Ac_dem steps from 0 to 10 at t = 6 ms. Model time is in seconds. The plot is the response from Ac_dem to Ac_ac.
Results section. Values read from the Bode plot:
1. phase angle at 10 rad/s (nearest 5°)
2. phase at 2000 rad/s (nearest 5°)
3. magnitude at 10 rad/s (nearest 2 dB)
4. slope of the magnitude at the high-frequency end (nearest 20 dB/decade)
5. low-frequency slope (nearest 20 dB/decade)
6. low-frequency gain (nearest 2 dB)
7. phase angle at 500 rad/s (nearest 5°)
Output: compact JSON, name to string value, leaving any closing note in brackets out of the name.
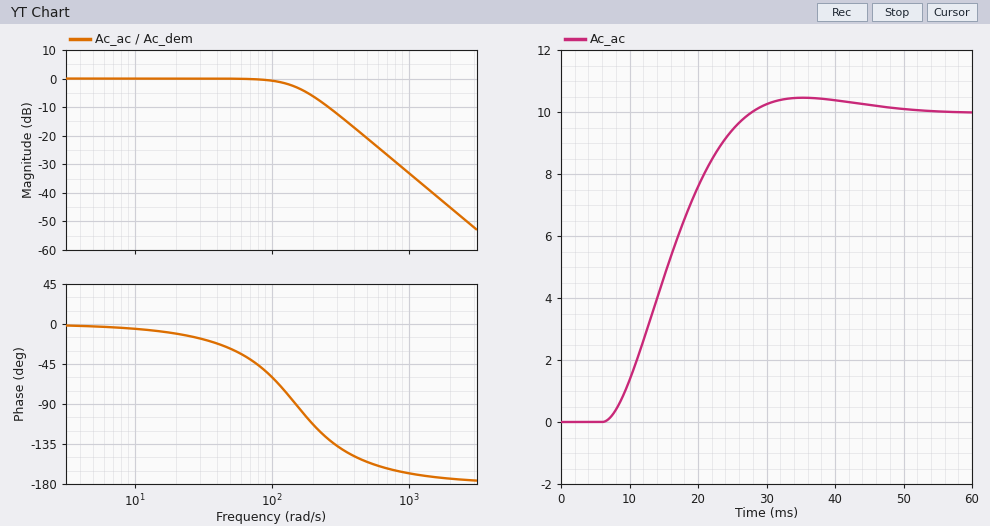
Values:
{"phase angle at 10 rad/s": "-5°", "phase at 2000 rad/s": "-175°", "magnitude at 10 rad/s": "0 dB", "slope of the magnitude at the high-frequency end": "-40 dB/decade", "low-frequency slope": "0 dB/decade", "low-frequency gain": "0 dB", "phase angle at 500 rad/s": "-155°"}
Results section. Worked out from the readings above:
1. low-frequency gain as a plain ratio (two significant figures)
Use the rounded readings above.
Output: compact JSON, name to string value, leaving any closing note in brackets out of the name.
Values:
{"low-frequency gain as a plain ratio": "1.0"}
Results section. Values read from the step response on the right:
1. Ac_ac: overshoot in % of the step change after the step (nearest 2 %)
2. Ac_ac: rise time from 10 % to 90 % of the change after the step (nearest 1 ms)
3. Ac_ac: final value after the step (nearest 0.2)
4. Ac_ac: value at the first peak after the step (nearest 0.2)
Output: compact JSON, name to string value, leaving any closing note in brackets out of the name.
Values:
{"Ac_ac: overshoot in % of the step change after the step": "4 %", "Ac_ac: rise time from 10 % to 90 % of the change after the step": "14 ms", "Ac_ac: final value after the step": "10.0", "Ac_ac: value at the first peak after the step": "10.4"}
